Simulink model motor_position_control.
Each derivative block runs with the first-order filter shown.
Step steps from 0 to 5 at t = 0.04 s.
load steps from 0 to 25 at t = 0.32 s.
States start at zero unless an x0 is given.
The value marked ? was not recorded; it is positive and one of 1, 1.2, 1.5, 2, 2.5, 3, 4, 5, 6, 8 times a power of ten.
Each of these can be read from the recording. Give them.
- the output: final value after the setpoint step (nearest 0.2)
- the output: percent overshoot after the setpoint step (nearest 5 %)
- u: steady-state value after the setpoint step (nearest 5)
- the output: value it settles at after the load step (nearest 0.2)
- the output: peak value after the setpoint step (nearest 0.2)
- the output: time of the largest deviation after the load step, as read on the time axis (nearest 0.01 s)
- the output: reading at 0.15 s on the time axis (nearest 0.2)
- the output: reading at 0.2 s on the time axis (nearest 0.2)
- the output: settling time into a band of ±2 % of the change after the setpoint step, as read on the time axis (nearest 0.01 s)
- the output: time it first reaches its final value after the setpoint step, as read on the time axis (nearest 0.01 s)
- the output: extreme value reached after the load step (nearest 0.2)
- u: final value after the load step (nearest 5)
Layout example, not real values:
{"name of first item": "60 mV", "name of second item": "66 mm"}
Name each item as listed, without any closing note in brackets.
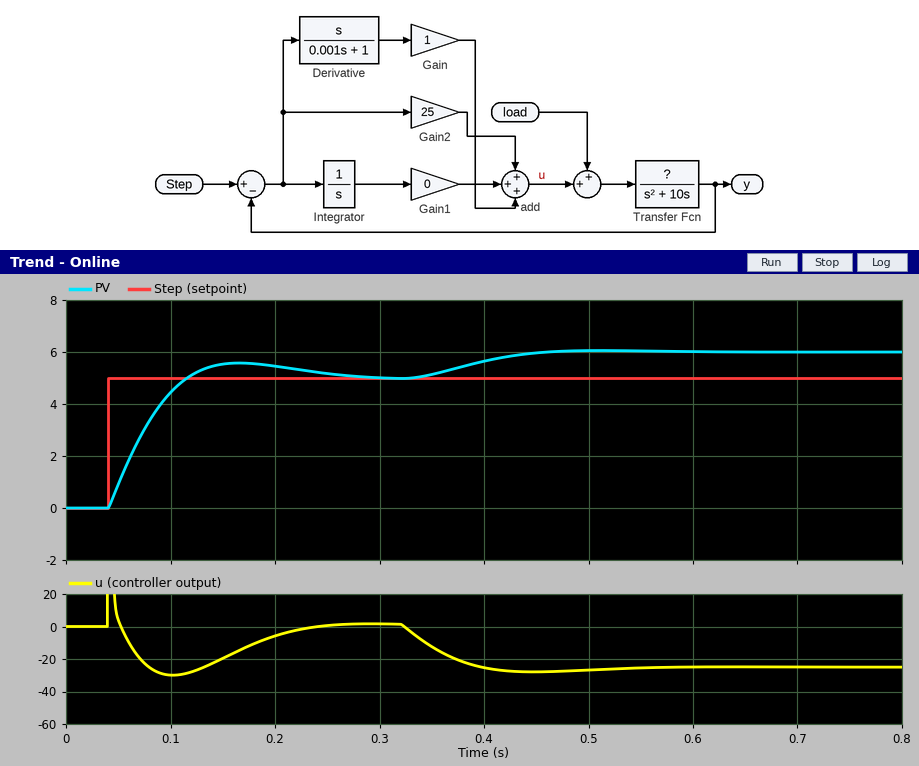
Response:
{"the output: final value after the setpoint step": "5.0", "the output: percent overshoot after the setpoint step": "10 %", "u: steady-state value after the setpoint step": "0", "the output: value it settles at after the load step": "6.0", "the output: peak value after the setpoint step": "5.6", "the output: time of the largest deviation after the load step, as read on the time axis": "0.51 s", "the output: reading at 0.15 s on the time axis": "5.6", "the output: reading at 0.2 s on the time axis": "5.4", "the output: settling time into a band of ±2 % of the change after the setpoint step, as read on the time axis": "0.27 s", "the output: time it first reaches its final value after the setpoint step, as read on the time axis": "0.12 s", "the output: extreme value reached after the load step": "6.0", "u: final value after the load step": "-25"}
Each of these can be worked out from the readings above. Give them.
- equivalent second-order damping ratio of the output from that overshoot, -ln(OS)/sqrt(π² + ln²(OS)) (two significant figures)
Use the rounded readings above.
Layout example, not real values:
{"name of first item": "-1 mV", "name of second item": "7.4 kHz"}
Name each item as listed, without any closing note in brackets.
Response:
{"equivalent second-order damping ratio of the output from that overshoot, -ln(OS)/sqrt(π² + ln²(OS))": "0.59"}
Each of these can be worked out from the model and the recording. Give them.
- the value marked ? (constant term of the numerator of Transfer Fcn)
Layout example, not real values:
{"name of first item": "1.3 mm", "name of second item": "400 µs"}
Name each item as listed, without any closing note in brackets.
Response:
{"the value marked ?": "20"}
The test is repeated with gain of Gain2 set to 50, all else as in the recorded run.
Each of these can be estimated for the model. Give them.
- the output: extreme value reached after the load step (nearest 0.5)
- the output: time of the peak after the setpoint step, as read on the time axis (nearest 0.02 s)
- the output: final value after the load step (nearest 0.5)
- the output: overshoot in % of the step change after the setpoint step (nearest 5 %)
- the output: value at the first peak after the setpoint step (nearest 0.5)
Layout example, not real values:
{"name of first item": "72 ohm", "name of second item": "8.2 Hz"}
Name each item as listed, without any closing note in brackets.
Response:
{"the output: extreme value reached after the load step": "5.5", "the output: time of the peak after the setpoint step, as read on the time axis": "0.12 s", "the output: final value after the load step": "5.5", "the output: overshoot in % of the step change after the setpoint step": "25 %", "the output: value at the first peak after the setpoint step": "6.0"}
